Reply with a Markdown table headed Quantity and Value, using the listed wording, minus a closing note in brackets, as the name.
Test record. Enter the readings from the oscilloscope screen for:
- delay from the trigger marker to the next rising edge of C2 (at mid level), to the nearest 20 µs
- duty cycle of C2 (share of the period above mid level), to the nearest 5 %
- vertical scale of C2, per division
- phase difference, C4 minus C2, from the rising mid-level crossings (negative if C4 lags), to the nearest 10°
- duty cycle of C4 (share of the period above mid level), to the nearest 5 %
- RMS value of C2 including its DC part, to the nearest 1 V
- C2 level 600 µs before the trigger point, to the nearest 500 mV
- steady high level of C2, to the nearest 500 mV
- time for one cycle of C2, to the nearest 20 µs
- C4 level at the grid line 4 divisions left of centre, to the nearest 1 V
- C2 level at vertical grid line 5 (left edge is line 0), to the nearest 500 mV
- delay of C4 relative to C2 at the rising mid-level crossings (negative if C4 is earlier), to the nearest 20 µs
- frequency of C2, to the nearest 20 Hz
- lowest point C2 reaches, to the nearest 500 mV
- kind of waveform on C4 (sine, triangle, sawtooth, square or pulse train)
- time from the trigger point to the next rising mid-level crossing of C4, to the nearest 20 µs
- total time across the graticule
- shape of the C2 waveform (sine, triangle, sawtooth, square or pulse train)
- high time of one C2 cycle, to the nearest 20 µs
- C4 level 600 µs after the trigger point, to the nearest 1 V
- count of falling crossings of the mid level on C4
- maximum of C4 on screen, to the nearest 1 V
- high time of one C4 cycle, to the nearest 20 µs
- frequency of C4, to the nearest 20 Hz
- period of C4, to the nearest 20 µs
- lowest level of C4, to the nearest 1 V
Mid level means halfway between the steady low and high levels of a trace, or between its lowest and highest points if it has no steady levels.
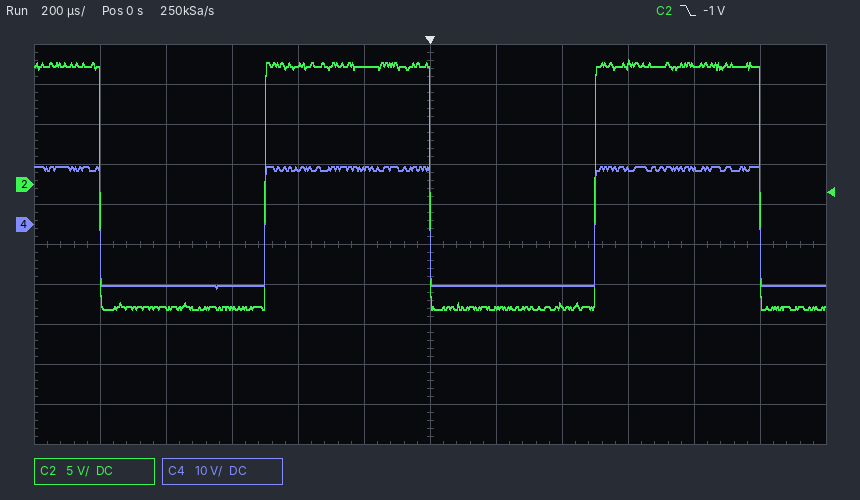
| Quantity | Value |
|---|---|
| delay from the trigger marker to the next rising edge of C2 (at mid level), to the nearest 20 µs | 500 µs |
| duty cycle of C2 (share of the period above mid level), to the nearest 5 % | 50 % |
| vertical scale of C2, per division | 5 V |
| phase difference, C4 minus C2, from the rising mid-level crossings (negative if C4 lags), to the nearest 10° | 0° |
| duty cycle of C4 (share of the period above mid level), to the nearest 5 % | 50 % |
| RMS value of C2 including its DC part, to the nearest 1 V | 15 V |
| C2 level 600 µs before the trigger point, to the nearest 500 mV | -15.5 V |
| steady high level of C2, to the nearest 500 mV | 15.0 V |
| time for one cycle of C2, to the nearest 20 µs | 1.00 ms |
| C4 level at the grid line 4 divisions left of centre, to the nearest 1 V | -15 V |
| C2 level at vertical grid line 5 (left edge is line 0), to the nearest 500 mV | 15.0 V |
| delay of C4 relative to C2 at the rising mid-level crossings (negative if C4 is earlier), to the nearest 20 µs | 0 µs |
| frequency of C2, to the nearest 20 Hz | 1.00 kHz |
| lowest point C2 reaches, to the nearest 500 mV | -15.5 V |
| kind of waveform on C4 | square |
| time from the trigger point to the next rising mid-level crossing of C4, to the nearest 20 µs | 500 µs |
| total time across the graticule | 2.4 ms |
| shape of the C2 waveform | square |
| high time of one C2 cycle, to the nearest 20 µs | 500 µs |
| C4 level 600 µs after the trigger point, to the nearest 1 V | 14 V |
| count of falling crossings of the mid level on C4 | 3 |
| maximum of C4 on screen, to the nearest 1 V | 14 V |
| high time of one C4 cycle, to the nearest 20 µs | 500 µs |
| frequency of C4, to the nearest 20 Hz | 1.00 kHz |
| period of C4, to the nearest 20 µs | 1.00 ms |
| lowest level of C4, to the nearest 1 V | -16 V |
